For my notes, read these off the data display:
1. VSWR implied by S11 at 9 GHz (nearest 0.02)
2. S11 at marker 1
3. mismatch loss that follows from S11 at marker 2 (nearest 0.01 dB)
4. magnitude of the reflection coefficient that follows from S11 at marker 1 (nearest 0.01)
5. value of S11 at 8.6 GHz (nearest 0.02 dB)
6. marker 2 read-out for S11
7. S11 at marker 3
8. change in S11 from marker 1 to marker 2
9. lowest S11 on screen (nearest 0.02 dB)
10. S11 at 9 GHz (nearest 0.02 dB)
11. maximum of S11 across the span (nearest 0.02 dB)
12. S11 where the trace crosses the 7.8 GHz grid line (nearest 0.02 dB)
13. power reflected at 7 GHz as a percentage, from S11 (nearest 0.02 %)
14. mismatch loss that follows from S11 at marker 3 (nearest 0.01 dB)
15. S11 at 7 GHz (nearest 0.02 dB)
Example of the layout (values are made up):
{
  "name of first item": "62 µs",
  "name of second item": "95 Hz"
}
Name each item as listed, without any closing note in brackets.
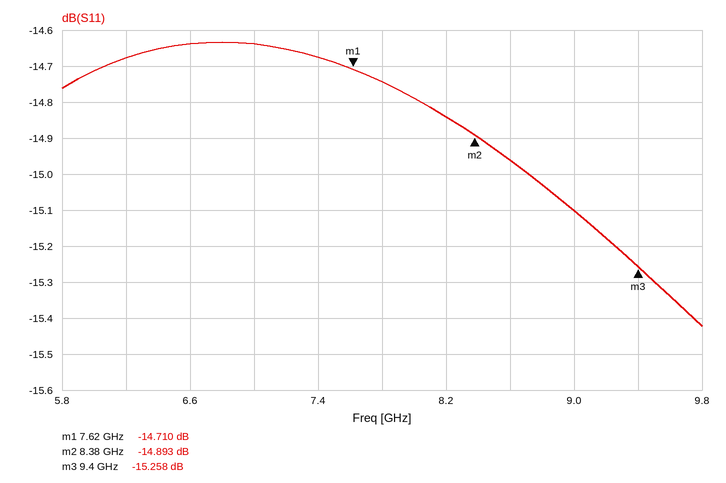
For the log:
{
  "VSWR implied by S11 at 9 GHz": "1.42",
  "S11 at marker 1": "-14.710 dB",
  "mismatch loss that follows from S11 at marker 2": "0.14 dB",
  "magnitude of the reflection coefficient that follows from S11 at marker 1": "0.18",
  "value of S11 at 8.6 GHz": "-14.96 dB",
  "marker 2 read-out for S11": "-14.893 dB",
  "S11 at marker 3": "-15.258 dB",
  "change in S11 from marker 1 to marker 2": "-0.183 dB",
  "lowest S11 on screen": "-15.42 dB",
  "S11 at 9 GHz": "-15.10 dB",
  "maximum of S11 across the span": "-14.64 dB",
  "S11 where the trace crosses the 7.8 GHz grid line": "-14.74 dB",
  "power reflected at 7 GHz as a percentage, from S11": "3.44 %",
  "mismatch loss that follows from S11 at marker 3": "0.13 dB",
  "S11 at 7 GHz": "-14.64 dB"
}
